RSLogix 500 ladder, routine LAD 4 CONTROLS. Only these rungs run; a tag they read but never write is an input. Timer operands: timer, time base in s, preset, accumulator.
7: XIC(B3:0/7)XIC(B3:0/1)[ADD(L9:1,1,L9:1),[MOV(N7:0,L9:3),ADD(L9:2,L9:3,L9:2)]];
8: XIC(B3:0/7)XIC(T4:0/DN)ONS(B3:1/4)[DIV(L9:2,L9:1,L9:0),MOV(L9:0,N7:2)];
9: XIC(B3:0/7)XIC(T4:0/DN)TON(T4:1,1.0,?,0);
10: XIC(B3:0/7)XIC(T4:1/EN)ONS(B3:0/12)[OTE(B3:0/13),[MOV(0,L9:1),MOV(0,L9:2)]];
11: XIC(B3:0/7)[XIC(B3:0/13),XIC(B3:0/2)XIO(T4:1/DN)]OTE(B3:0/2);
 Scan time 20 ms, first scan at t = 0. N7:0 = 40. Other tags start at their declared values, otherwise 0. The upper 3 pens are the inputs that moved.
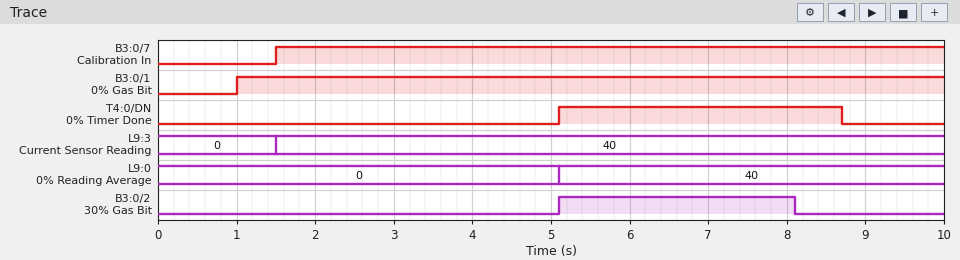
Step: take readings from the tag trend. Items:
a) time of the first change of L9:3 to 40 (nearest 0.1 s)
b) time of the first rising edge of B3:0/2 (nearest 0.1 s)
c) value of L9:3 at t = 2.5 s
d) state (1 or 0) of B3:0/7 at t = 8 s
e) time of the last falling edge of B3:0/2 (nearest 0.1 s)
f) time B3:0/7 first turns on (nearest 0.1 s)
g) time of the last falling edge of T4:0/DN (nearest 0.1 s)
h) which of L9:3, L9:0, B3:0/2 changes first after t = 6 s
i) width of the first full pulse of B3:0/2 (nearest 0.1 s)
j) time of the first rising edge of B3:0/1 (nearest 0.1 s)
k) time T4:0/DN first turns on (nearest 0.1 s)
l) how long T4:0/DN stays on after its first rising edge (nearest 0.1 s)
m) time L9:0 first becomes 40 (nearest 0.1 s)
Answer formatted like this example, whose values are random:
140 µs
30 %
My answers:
1.5 s
5.1 s
40
1
8.1 s
1.5 s
8.7 s
B3:0/2
3.0 s
1.0 s
5.1 s
3.6 s
5.1 s
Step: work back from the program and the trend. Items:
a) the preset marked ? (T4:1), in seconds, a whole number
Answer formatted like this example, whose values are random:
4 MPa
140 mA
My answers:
3 s
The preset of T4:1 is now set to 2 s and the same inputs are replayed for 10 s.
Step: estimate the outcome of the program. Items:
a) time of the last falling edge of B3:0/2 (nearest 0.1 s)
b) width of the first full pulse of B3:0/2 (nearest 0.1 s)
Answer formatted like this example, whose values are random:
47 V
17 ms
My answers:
7.1 s
2.0 s
